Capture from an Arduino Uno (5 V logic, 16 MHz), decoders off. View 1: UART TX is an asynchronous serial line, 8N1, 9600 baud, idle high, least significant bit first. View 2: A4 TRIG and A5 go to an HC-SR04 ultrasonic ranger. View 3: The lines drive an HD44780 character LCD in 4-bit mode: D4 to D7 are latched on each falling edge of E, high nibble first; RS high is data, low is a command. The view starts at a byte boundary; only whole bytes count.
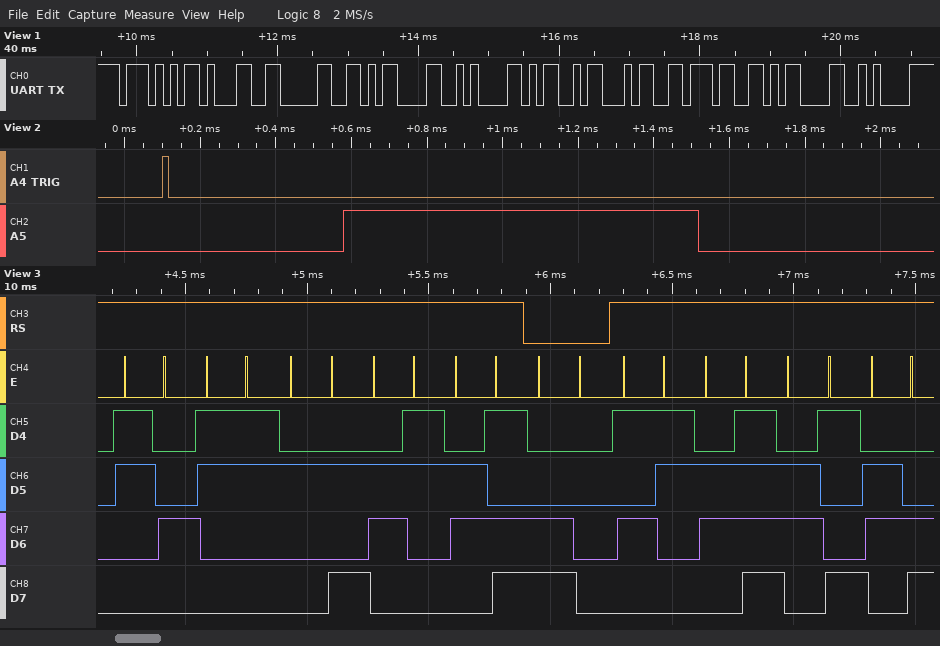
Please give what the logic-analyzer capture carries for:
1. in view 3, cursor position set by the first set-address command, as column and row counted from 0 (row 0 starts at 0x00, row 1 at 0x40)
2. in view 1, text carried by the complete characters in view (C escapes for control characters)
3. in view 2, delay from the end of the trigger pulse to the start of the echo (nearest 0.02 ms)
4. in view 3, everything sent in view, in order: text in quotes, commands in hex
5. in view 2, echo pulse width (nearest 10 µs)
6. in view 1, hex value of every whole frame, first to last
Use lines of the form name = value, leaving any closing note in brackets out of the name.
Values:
in view 3, cursor position set by the first set-address command, as column and row counted from 0 = column 0, row 1
in view 1, text carried by the complete characters in view = "W10\r\nM47\r\n"
in view 2, delay from the end of the trigger pulse to the start of the echo = 0.46 ms
in view 3, everything sent in view, in order: text in quotes, commands in hex = "43*cm" 0xC0 "Soil"
in view 2, echo pulse width = 940 µs
in view 1, hex value of every whole frame, first to last = 57 31 30 0D 0A 4D 34 37 0D 0A
